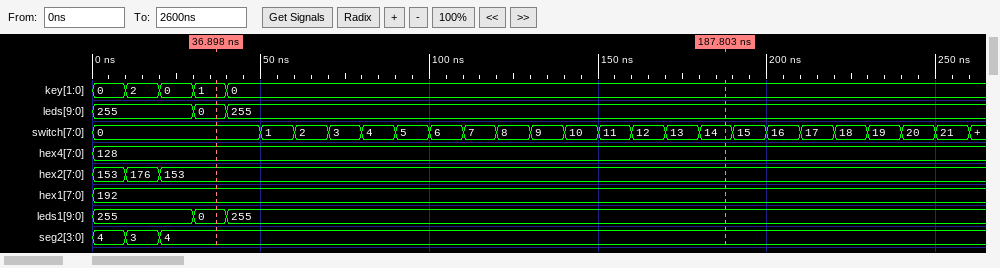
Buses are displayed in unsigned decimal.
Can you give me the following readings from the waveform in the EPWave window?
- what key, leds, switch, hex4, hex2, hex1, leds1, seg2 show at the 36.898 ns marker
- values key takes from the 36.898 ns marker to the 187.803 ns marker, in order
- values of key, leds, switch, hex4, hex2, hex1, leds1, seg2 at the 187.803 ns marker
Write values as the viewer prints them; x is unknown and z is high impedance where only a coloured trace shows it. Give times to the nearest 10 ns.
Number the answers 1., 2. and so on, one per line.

1. key=1, leds=0, switch=0, hex4=128, hex2=153, hex1=192, leds1=0, seg2=4
2. 1, 0
3. key=0, leds=255, switch=14, hex4=128, hex2=153, hex1=192, leds1=255, seg2=4
